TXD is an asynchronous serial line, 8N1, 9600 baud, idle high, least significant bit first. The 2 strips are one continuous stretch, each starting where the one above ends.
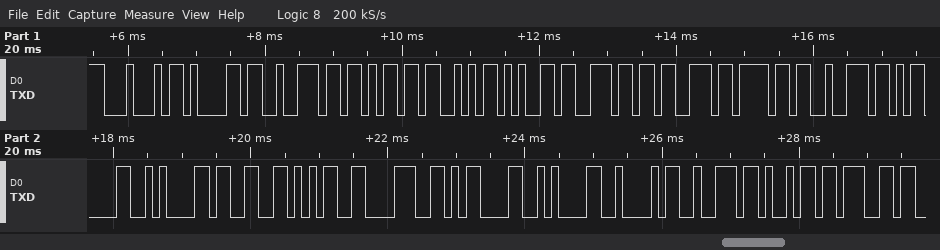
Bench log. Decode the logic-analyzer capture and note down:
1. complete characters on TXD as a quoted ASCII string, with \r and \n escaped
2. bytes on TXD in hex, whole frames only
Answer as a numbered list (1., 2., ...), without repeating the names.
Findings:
1. "DarkSensor\r\n358\r\nBrig"
2. 44 61 72 6B 53 65 6E 73 6F 72 0D 0A 33 35 38 0D 0A 42 72 69 67
